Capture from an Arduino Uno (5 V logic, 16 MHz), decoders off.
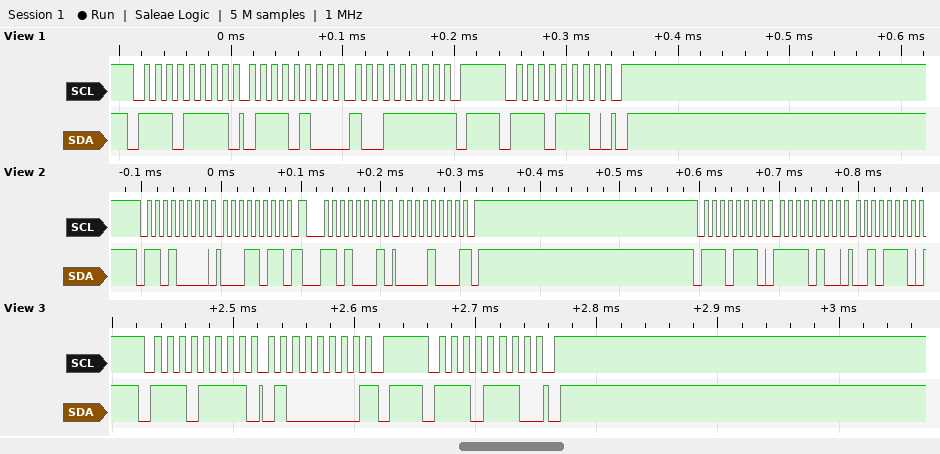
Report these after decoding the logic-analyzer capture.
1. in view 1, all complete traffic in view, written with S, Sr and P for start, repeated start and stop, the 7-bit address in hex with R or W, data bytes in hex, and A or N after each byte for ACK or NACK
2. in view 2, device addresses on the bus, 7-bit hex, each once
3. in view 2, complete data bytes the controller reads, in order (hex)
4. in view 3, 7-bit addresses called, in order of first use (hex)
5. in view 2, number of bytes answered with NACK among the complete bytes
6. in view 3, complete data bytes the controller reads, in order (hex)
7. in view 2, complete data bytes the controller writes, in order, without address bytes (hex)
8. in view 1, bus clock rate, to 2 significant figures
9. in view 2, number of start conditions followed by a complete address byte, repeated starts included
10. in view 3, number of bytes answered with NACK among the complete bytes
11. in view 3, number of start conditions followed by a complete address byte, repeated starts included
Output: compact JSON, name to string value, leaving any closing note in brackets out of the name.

{"in view 1, all complete traffic in view, written with S, Sr and P for start, repeated start and stop, the 7-bit address in hex with R or W, data bytes in hex, and A or N after each byte for ACK or NACK": "S 77R A 74 A 9F N P S 77W A P", "in view 2, device addresses on the bus, 7-bit hex, each once": "0x68 0x77", "in view 2, complete data bytes the controller reads, in order": "08", "in view 3, 7-bit addresses called, in order of first use": "0x77", "in view 2, number of bytes answered with NACK among the complete bytes": "1", "in view 3, complete data bytes the controller reads, in order": "40", "in view 2, complete data bytes the controller writes, in order, without address bytes": "1B F4 2E", "in view 1, bus clock rate, to 2 significant figures": "100 kHz", "in view 2, number of start conditions followed by a complete address byte, repeated starts included": "3", "in view 3, number of bytes answered with NACK among the complete bytes": "1", "in view 3, number of start conditions followed by a complete address byte, repeated starts included": "2"}
